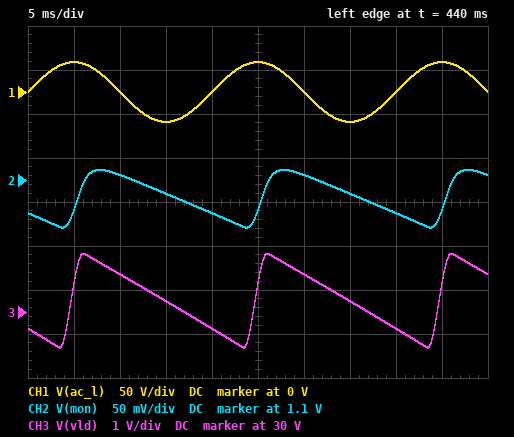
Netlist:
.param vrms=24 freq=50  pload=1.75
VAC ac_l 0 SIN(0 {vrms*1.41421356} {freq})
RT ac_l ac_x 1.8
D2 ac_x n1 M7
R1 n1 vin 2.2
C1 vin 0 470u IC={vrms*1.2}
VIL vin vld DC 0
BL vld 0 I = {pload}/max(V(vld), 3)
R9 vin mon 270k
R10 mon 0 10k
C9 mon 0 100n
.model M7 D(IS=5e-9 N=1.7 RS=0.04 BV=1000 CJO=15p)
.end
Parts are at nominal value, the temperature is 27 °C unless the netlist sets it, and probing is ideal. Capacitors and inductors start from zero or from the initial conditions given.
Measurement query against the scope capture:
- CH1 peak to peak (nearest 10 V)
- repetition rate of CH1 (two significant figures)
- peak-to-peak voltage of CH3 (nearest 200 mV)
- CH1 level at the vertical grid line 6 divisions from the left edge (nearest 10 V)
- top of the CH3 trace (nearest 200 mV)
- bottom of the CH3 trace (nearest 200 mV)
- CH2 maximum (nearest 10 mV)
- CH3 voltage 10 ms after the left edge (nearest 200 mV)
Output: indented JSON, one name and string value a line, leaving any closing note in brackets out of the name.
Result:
{
  "CH1 peak to peak": "70 V",
  "repetition rate of CH1": "50 Hz",
  "peak-to-peak voltage of CH3": "2.2 V",
  "CH1 level at the vertical grid line 6 divisions from the left edge": "0 V",
  "top of the CH3 trace": "31.4 V",
  "bottom of the CH3 trace": "29.2 V",
  "CH2 maximum": "1.11 V",
  "CH3 voltage 10 ms after the left edge": "30.8 V"
}
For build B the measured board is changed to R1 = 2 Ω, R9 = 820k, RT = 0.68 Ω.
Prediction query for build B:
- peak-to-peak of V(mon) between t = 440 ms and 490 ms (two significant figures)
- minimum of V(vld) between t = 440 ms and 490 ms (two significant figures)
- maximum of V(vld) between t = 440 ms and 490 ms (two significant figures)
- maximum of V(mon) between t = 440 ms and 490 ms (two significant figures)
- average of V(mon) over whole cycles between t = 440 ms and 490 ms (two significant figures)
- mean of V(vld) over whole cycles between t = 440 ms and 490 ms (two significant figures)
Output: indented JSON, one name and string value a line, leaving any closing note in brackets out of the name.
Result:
{
  "peak-to-peak of V(mon) between t = 440 ms and 490 ms": "22 mV",
  "minimum of V(vld) between t = 440 ms and 490 ms": "30 V",
  "maximum of V(vld) between t = 440 ms and 490 ms": "32 V",
  "maximum of V(mon) between t = 440 ms and 490 ms": "380 mV",
  "average of V(mon) over whole cycles between t = 440 ms and 490 ms": "370 mV",
  "mean of V(vld) over whole cycles between t = 440 ms and 490 ms": "31 V"
}
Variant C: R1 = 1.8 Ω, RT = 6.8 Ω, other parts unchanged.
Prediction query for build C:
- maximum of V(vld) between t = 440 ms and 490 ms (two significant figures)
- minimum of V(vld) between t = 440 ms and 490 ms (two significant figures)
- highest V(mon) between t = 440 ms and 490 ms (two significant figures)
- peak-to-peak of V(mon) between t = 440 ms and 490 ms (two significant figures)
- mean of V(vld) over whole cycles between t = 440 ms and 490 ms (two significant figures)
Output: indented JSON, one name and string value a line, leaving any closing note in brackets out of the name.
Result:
{
  "maximum of V(vld) between t = 440 ms and 490 ms": "29 V",
  "minimum of V(vld) between t = 440 ms and 490 ms": "27 V",
  "highest V(mon) between t = 440 ms and 490 ms": "1.0 V",
  "peak-to-peak of V(mon) between t = 440 ms and 490 ms": "68 mV",
  "mean of V(vld) over whole cycles between t = 440 ms and 490 ms": "28 V"
}
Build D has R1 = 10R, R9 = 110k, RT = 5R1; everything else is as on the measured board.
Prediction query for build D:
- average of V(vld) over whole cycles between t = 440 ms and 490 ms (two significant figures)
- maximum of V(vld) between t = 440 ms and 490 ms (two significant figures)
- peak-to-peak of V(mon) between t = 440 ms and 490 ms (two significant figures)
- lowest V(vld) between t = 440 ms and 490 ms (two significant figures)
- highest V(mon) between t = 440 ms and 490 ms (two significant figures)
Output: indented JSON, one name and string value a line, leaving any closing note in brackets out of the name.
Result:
{
  "average of V(vld) over whole cycles between t = 440 ms and 490 ms": "26 V",
  "maximum of V(vld) between t = 440 ms and 490 ms": "27 V",
  "peak-to-peak of V(mon) between t = 440 ms and 490 ms": "170 mV",
  "lowest V(vld) between t = 440 ms and 490 ms": "25 V",
  "highest V(mon) between t = 440 ms and 490 ms": "2.2 V"
}
